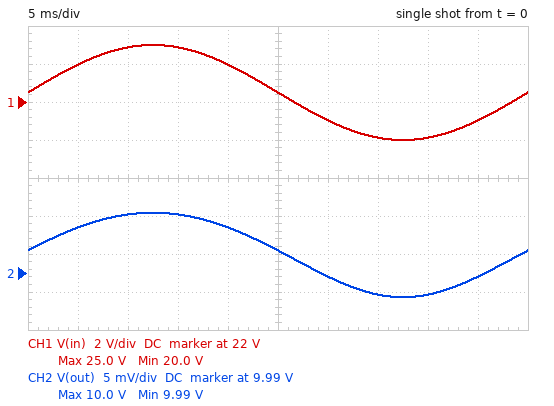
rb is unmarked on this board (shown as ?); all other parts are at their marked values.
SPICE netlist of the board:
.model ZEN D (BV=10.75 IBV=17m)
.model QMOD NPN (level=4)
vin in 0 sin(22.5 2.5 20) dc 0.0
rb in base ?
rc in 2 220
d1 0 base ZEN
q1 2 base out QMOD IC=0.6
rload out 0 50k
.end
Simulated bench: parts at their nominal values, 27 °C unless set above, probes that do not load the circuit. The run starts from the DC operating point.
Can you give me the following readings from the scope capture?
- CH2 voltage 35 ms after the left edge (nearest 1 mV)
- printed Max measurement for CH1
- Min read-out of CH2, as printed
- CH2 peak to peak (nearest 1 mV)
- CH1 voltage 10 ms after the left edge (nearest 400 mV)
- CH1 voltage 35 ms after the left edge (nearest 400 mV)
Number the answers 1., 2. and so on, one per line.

1. 9.987 V
2. 25.0 V
3. 9.99 V
4. 11 mV
5. 24.8 V
6. 20.0 V
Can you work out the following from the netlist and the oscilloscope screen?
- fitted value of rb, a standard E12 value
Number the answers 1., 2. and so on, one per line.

1. 1.8 kΩ
